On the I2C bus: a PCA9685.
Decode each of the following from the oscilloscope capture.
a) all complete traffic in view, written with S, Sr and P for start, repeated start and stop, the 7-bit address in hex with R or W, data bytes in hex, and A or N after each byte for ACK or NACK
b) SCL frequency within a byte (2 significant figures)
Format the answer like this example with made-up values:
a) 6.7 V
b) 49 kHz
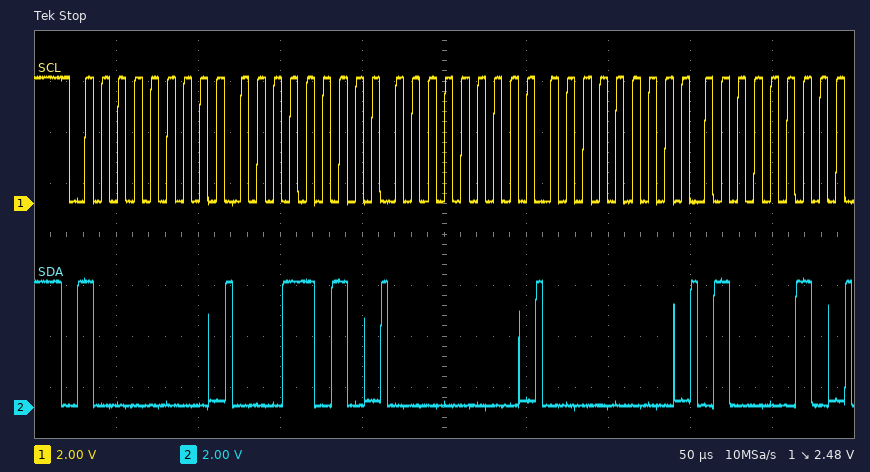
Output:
a) S 40W A 1A A 00 A 00 A 42 A
b) 100 kHz
